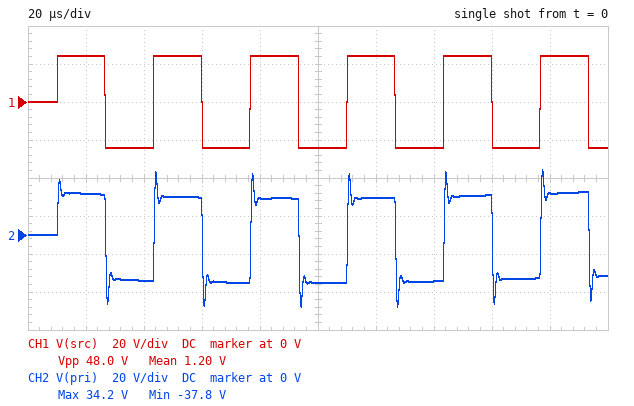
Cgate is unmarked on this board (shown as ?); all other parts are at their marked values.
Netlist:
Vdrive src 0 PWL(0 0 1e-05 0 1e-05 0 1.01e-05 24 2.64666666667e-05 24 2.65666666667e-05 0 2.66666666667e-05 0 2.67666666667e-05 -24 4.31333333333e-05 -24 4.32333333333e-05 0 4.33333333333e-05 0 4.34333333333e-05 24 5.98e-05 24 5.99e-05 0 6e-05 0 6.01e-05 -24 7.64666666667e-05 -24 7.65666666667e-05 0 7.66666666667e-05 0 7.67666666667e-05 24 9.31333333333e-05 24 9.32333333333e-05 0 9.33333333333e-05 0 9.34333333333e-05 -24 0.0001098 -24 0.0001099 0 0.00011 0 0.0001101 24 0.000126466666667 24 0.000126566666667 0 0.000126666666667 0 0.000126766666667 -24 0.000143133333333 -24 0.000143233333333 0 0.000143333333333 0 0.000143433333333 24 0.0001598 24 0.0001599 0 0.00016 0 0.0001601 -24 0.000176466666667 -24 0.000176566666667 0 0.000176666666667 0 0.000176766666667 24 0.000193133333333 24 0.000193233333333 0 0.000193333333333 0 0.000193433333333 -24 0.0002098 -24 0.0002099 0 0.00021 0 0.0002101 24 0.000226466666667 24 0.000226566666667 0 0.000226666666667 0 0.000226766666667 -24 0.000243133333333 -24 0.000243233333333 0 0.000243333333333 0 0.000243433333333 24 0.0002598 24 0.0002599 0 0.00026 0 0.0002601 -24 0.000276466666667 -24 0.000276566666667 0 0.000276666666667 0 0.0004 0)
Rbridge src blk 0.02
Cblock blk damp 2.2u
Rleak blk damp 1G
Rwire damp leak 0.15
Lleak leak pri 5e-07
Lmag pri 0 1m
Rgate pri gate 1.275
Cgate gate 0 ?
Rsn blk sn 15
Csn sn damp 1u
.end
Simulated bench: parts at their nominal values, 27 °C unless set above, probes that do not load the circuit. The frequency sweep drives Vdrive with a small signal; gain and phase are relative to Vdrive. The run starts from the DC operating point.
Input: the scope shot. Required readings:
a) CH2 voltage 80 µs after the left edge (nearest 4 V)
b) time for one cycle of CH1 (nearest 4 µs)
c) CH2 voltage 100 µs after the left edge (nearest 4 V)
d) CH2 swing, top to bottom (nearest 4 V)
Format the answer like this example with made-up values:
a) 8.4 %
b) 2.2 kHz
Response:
a) 20 V
b) 32 µs
c) -24 V
d) 72 V
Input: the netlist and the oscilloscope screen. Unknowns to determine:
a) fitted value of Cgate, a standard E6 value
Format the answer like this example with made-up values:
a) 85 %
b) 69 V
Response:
a) 220 nF
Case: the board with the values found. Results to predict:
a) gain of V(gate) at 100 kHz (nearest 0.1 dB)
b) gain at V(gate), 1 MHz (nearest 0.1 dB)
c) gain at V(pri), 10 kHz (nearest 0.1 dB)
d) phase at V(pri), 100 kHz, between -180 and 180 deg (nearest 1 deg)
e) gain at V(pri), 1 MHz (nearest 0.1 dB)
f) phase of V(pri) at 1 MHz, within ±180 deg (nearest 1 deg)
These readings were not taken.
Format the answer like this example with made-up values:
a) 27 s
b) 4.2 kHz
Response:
a) -0.6 dB
b) -11.6 dB
c) 0.1 dB
d) -1 deg
e) -5.5 dB
f) -88 deg
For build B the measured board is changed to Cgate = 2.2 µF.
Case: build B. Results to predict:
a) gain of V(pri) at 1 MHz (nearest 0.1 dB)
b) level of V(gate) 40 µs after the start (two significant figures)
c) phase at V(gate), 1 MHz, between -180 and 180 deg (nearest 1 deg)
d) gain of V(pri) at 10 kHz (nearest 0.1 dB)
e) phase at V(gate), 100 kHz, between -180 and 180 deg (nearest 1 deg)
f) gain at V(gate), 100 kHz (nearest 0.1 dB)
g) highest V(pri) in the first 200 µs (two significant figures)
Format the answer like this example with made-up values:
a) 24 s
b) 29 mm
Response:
a) -8.3 dB
b) -13 V
c) -154 deg
d) -4.6 dB
e) -53 deg
f) -8.2 dB
g) 25 V
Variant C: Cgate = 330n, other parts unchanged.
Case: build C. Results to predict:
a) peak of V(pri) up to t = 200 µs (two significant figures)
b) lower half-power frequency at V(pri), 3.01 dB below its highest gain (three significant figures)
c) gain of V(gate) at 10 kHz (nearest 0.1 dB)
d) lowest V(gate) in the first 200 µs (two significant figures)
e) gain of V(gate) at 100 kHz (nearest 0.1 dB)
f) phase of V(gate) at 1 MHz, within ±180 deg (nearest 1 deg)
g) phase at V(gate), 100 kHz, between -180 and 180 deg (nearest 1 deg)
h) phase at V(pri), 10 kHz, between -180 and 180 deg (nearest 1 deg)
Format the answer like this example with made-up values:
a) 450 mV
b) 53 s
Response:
a) 31 V
b) 2.60 kHz
c) -0.2 dB
d) -29 V
e) -1.0 dB
f) -151 deg
g) -16 deg
h) 0 deg
